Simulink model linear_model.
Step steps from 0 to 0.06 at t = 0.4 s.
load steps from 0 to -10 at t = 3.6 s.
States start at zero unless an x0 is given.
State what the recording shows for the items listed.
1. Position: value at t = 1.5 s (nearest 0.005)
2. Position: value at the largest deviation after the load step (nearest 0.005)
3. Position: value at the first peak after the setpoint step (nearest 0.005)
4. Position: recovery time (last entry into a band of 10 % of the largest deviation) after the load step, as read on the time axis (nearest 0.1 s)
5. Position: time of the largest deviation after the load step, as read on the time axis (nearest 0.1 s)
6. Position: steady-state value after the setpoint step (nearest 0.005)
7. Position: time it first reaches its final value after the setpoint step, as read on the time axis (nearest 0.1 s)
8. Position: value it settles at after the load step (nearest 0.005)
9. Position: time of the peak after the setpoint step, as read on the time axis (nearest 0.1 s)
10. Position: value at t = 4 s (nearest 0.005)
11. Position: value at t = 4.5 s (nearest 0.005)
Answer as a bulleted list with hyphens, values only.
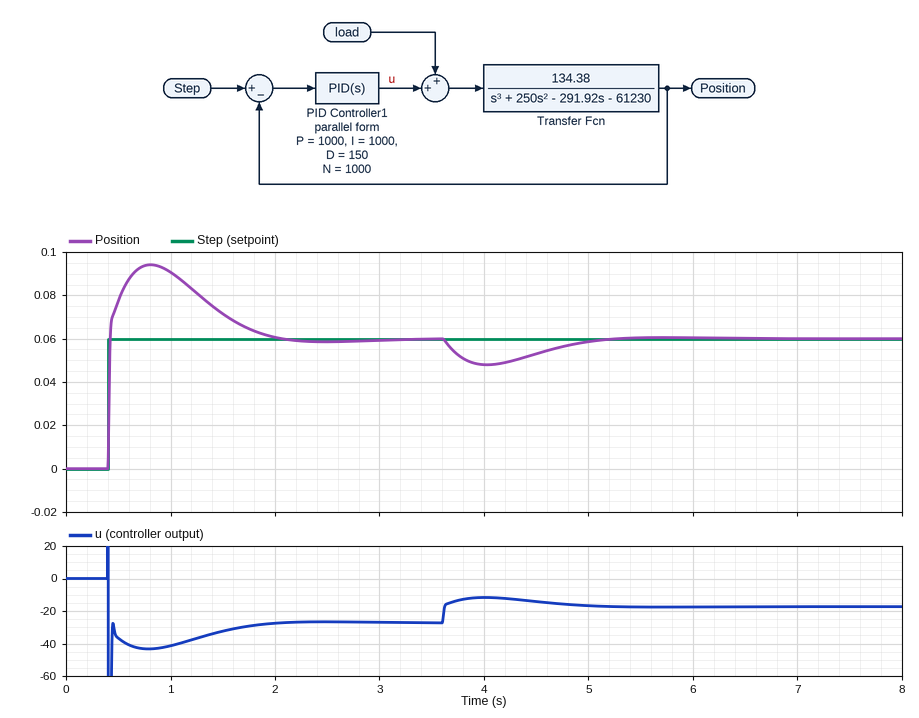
- 0.070
- 0.050
- 0.095
- 5.0 s
- 4.0 s
- 0.060
- 0.4 s
- 0.060
- 0.8 s
- 0.050
- 0.055
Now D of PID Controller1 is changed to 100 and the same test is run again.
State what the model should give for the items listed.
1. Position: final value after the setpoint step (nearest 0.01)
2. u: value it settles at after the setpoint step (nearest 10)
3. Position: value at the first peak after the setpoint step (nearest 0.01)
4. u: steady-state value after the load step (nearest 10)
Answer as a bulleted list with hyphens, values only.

- 0.06
- -30
- 0.10
- -20
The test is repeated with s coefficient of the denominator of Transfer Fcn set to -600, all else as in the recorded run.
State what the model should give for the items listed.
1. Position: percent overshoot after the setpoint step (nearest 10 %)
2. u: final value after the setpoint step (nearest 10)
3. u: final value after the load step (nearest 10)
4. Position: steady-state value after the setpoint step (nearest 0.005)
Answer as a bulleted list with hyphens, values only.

- 60 %
- -30
- -20
- 0.060
